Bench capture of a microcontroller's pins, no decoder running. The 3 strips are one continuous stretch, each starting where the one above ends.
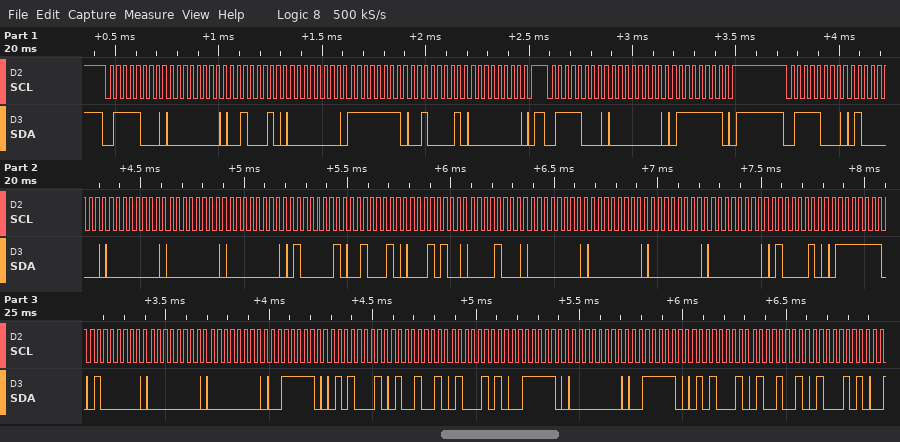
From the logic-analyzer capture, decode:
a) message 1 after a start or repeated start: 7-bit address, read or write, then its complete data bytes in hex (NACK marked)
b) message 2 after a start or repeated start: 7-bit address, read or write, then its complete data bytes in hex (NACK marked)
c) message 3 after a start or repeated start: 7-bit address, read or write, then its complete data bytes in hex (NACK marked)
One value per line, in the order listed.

0x3C write: 00 22 00 FF 21 00
0x3C write: 00 7F
0x3C write: 40 00 00 00 41 22 14 08 00 00 00 00 42 7F 40 00 00 3E 51 49 45 3E 00 3E 51 49 45
